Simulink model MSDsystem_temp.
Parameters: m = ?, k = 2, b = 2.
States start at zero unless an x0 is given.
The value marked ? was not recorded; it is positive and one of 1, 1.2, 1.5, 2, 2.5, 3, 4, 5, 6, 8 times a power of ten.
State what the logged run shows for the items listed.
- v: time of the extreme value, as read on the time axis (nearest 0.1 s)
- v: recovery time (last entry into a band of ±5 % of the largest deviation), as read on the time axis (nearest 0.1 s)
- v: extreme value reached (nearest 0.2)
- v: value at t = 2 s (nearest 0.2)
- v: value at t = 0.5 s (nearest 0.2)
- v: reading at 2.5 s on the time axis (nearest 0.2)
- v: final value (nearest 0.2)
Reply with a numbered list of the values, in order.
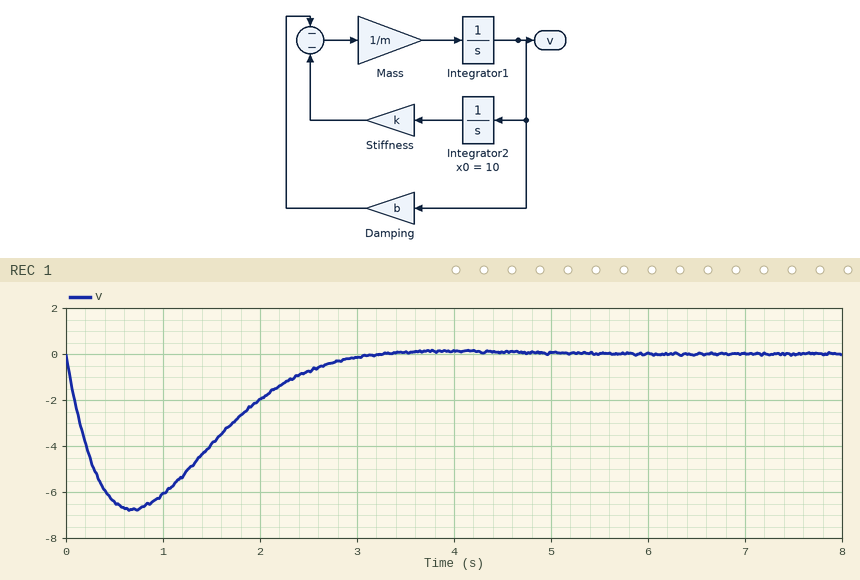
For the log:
1. 0.7 s
2. 2.8 s
3. -6.8
4. -2.0
5. -6.4
6. -0.8
7. 0.0
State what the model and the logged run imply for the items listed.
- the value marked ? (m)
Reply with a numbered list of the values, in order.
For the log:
1. 0.8
